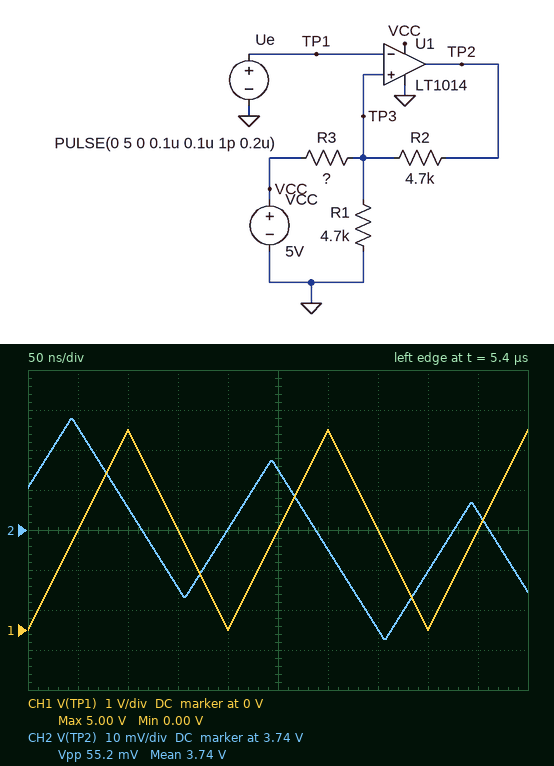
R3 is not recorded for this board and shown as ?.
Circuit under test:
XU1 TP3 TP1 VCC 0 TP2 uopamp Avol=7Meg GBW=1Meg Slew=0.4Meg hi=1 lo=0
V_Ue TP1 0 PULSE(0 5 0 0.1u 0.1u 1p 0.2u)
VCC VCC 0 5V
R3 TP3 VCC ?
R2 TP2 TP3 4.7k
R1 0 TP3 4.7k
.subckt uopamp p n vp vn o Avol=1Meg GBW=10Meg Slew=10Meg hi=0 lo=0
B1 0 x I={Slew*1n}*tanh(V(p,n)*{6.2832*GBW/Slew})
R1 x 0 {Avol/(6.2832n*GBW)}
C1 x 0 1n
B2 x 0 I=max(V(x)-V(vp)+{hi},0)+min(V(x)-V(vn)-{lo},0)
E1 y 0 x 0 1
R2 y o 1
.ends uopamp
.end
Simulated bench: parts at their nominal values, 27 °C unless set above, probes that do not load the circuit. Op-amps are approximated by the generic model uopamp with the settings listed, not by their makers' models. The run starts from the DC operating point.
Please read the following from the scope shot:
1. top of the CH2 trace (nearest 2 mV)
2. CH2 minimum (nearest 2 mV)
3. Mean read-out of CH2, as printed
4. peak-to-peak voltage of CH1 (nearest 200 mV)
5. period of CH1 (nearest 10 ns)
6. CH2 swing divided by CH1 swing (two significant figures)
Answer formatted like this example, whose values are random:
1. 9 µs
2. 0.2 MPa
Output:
1. 3.768 V
2. 3.712 V
3. 3.74 V
4. 5.0 V
5. 200 ns
6. 0.011
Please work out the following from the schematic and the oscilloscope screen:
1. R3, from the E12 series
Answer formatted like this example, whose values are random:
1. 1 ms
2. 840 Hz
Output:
1. 22 kΩ
